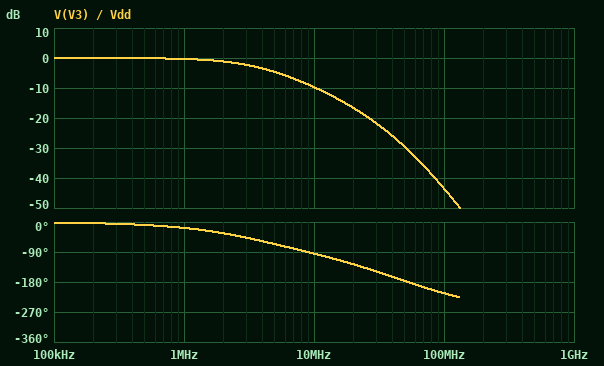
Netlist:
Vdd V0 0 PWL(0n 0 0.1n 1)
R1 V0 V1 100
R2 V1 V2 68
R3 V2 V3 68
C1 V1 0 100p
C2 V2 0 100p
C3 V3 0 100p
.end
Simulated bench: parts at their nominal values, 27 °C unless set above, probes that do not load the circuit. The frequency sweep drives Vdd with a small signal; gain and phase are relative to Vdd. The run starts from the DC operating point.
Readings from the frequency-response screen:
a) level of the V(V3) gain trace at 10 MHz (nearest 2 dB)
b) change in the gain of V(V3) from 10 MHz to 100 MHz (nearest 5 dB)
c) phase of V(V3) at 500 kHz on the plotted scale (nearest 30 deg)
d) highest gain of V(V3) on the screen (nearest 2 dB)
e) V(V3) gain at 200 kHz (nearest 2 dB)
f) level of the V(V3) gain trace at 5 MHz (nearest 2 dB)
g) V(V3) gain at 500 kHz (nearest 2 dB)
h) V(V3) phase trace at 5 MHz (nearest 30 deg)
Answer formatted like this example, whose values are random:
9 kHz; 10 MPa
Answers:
-10 dB; -35 dB; 0 deg; 0 dB; 0 dB; -4 dB; 0 dB; -60 deg
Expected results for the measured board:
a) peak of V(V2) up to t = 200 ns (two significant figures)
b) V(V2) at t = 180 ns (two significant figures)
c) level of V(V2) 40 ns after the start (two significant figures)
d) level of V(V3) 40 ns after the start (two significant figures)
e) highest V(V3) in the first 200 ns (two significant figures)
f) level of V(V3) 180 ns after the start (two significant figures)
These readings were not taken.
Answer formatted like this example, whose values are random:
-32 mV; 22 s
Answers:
990 mV; 980 mV; 600 mV; 530 mV; 990 mV; 980 mV
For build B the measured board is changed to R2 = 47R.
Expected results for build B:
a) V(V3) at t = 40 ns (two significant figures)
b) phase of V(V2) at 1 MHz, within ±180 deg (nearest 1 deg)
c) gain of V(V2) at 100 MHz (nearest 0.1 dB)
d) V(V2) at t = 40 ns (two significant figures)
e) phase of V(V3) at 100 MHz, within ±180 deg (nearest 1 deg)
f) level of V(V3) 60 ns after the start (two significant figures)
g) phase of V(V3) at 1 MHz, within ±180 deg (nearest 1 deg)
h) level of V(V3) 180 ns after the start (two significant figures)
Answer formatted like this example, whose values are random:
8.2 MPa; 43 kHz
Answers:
570 mV; -14 deg; -28.3 dB; 640 mV; 154 deg; 740 mV; -16 deg; 990 mV
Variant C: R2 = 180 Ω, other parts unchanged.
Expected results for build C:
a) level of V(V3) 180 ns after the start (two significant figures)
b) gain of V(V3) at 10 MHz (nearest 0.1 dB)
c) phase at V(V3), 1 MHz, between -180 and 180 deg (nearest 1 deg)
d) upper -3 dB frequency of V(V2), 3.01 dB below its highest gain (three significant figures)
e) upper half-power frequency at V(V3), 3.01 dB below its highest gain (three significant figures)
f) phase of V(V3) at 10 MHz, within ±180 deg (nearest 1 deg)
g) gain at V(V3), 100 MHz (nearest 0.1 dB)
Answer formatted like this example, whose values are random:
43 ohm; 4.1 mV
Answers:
930 mV; -13.1 dB; -25 deg; 2.51 MHz; 2.48 MHz; -109 deg; -51.0 dB
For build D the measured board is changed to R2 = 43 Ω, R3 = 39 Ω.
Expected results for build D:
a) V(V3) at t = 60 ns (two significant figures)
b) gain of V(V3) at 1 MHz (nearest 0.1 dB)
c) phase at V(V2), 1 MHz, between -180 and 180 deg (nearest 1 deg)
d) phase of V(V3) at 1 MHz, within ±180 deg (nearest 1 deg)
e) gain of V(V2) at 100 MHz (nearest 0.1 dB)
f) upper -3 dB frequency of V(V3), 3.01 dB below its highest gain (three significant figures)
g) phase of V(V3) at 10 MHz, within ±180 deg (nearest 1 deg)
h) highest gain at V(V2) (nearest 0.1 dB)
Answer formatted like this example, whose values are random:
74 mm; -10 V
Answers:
770 mV; -0.2 dB; -14 deg; -15 deg; -28.7 dB; 4.17 MHz; -84 deg; 0 dB
